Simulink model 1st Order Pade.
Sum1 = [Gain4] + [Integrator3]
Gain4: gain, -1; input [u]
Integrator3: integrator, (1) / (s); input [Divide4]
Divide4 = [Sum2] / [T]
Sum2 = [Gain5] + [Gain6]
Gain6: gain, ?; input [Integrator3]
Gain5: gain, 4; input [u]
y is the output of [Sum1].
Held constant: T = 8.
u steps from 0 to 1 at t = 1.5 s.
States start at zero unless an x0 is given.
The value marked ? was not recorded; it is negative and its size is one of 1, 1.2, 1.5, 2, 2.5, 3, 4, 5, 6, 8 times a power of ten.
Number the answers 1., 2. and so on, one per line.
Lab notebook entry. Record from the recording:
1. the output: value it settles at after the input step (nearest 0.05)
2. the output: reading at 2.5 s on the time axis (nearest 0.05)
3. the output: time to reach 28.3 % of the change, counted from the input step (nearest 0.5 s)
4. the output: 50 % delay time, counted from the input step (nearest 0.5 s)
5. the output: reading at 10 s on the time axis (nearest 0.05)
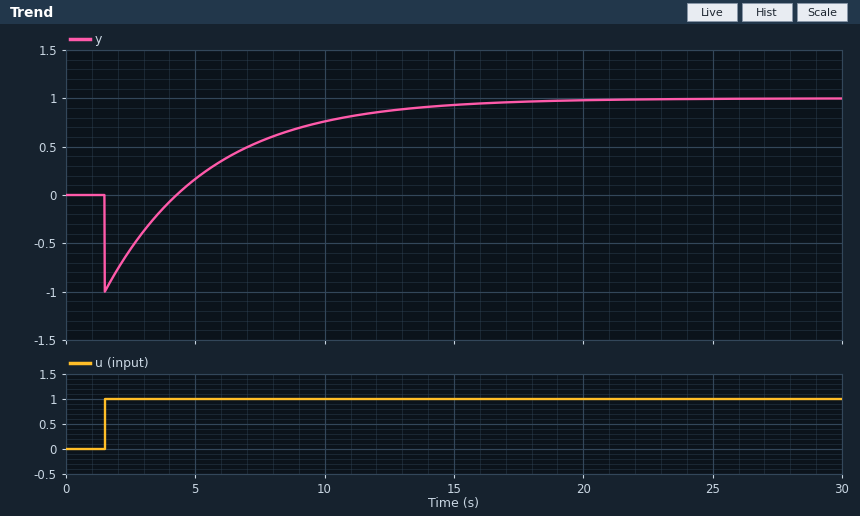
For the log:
1. 1.00
2. -0.55
3. 4.0 s
4. 5.5 s
5. 0.75
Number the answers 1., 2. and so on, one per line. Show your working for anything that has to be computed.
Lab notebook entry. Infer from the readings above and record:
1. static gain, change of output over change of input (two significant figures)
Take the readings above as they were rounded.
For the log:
1. (1 - 0) / (1 - 0) = 1.0
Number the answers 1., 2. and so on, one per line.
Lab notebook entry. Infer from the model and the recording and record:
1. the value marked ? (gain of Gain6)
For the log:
1. -2
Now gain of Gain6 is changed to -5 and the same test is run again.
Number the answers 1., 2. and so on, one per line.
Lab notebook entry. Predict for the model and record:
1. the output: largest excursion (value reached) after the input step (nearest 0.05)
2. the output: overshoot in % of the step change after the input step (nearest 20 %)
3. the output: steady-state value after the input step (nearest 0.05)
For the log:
1. -1.00
2. 400 %
3. -0.20
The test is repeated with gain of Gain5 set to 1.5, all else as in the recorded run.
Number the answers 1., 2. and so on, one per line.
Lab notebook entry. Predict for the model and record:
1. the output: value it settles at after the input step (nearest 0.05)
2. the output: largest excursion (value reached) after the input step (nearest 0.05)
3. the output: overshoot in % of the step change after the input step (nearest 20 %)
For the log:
1. -0.25
2. -1.00
3. 300 %
